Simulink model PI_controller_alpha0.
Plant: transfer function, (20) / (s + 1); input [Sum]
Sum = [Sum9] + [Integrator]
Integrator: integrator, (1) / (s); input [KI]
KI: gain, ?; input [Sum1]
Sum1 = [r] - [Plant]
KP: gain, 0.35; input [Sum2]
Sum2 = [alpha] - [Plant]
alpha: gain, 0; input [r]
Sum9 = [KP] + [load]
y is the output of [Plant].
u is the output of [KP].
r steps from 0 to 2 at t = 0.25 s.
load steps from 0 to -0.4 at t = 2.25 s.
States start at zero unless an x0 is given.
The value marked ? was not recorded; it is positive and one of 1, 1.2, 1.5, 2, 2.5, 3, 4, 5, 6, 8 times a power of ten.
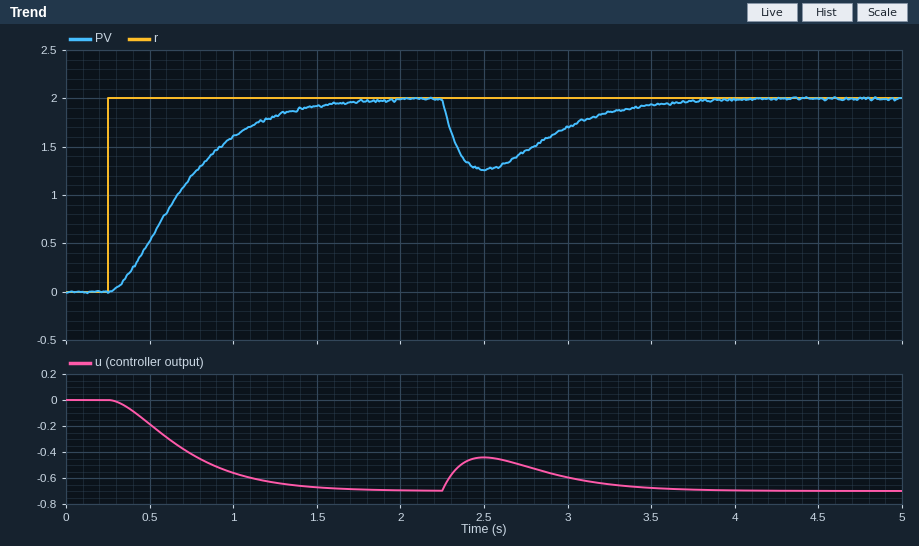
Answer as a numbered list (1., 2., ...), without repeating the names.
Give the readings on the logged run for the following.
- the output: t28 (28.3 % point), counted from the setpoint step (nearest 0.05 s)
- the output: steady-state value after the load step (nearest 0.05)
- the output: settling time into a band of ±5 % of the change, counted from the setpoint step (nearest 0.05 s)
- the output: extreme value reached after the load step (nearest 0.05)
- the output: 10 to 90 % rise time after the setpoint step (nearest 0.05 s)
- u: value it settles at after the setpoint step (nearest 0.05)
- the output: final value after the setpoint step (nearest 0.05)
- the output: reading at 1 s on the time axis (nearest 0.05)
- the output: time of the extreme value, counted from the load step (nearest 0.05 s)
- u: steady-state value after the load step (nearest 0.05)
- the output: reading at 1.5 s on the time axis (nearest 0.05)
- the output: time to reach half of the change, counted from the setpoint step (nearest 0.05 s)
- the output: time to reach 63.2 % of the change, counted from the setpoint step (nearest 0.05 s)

1. 0.25 s
2. 2.00
3. 1.20 s
4. 1.25
5. 0.85 s
6. -0.70
7. 2.00
8. 1.60
9. 0.25 s
10. -0.70
11. 1.90
12. 0.40 s
13. 0.55 s
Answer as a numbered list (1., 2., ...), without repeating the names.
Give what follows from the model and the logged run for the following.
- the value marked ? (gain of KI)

1. 0.8
